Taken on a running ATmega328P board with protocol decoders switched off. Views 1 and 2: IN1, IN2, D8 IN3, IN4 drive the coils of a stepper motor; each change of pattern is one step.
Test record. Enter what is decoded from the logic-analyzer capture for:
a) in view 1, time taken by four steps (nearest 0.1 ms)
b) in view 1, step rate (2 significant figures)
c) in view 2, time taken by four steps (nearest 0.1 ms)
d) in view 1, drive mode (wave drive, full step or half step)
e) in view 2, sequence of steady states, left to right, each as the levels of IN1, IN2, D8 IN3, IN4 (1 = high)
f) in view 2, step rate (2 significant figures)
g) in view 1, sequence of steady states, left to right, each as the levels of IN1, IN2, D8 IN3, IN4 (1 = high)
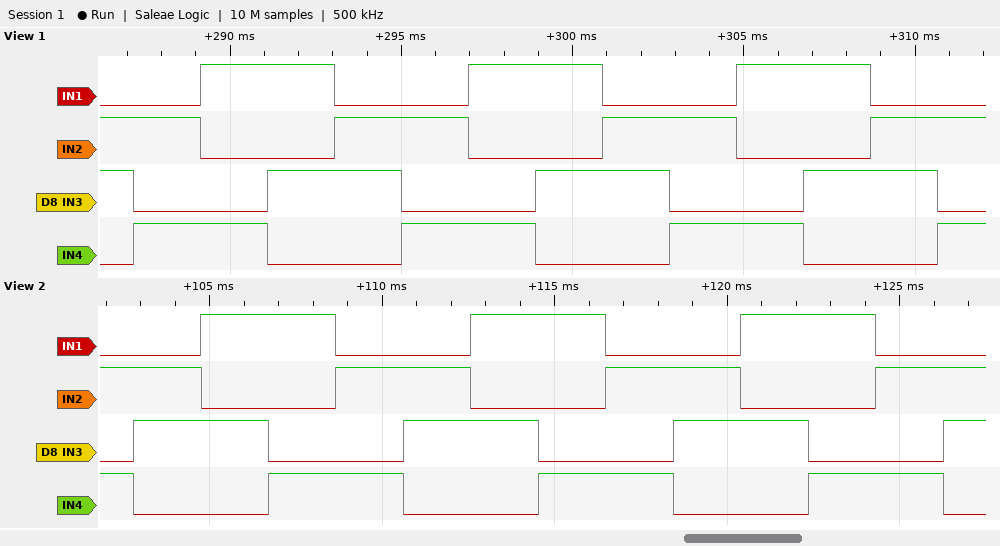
7.8 ms
510 steps/s
7.8 ms
full step
0101 0110 1010 1001 0101 0110 1010 1001 0101 0110 1010 1001 0101 0110
510 steps/s
0110 0101 1001 1010 0110 0101 1001 1010 0110 0101 1001 1010 0110 0101
